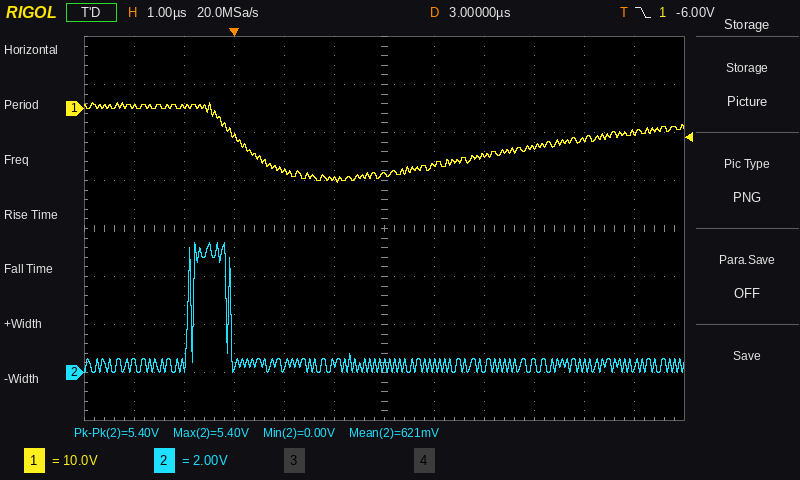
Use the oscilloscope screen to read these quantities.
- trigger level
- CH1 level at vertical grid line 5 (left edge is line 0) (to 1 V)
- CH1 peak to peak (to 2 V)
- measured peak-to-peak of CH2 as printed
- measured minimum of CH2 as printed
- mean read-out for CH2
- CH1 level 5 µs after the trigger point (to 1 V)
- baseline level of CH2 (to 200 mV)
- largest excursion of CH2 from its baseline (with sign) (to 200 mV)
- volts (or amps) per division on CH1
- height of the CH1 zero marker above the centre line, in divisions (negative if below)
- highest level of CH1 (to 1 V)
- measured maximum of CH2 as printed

-6.00 V
-15 V
16 V
5.40 V
0.00 V
621 mV
-10 V
400 mV
+5.0 V
10 V
+2.5 div
1 V
5.40 V
